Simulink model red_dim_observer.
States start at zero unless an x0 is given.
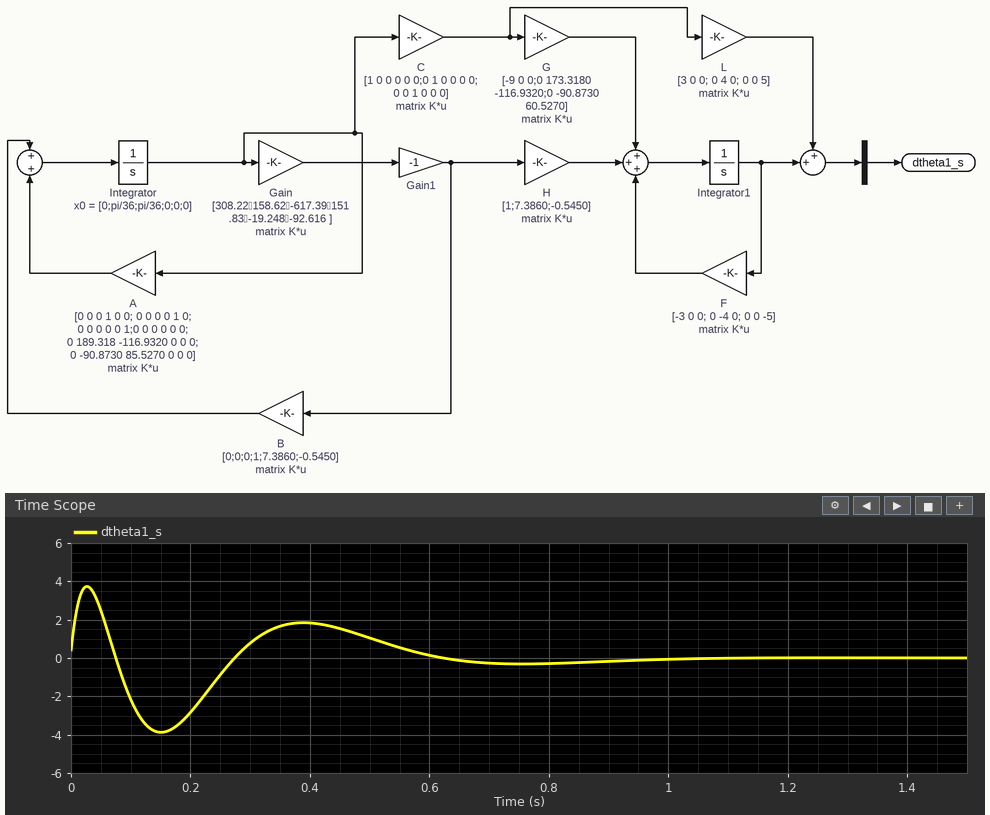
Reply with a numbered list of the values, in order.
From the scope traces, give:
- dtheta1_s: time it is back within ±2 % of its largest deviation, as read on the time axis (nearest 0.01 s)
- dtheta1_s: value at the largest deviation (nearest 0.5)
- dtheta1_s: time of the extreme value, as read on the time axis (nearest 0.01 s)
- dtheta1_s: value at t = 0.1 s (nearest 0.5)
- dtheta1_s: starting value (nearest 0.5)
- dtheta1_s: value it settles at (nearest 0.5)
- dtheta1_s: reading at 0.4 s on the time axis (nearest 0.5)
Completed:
1. 0.98 s
2. -4.0
3. 0.15 s
4. -2.0
5. 0.5
6. 0.0
7. 2.0
